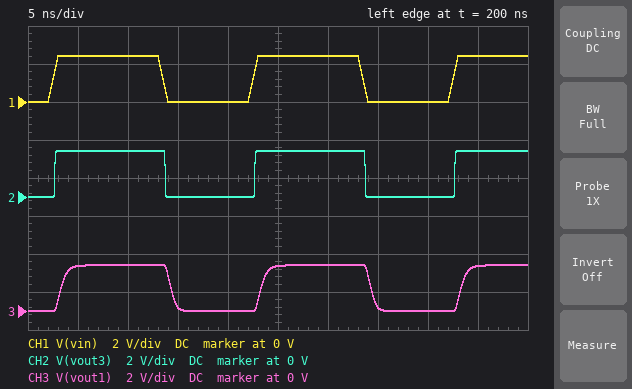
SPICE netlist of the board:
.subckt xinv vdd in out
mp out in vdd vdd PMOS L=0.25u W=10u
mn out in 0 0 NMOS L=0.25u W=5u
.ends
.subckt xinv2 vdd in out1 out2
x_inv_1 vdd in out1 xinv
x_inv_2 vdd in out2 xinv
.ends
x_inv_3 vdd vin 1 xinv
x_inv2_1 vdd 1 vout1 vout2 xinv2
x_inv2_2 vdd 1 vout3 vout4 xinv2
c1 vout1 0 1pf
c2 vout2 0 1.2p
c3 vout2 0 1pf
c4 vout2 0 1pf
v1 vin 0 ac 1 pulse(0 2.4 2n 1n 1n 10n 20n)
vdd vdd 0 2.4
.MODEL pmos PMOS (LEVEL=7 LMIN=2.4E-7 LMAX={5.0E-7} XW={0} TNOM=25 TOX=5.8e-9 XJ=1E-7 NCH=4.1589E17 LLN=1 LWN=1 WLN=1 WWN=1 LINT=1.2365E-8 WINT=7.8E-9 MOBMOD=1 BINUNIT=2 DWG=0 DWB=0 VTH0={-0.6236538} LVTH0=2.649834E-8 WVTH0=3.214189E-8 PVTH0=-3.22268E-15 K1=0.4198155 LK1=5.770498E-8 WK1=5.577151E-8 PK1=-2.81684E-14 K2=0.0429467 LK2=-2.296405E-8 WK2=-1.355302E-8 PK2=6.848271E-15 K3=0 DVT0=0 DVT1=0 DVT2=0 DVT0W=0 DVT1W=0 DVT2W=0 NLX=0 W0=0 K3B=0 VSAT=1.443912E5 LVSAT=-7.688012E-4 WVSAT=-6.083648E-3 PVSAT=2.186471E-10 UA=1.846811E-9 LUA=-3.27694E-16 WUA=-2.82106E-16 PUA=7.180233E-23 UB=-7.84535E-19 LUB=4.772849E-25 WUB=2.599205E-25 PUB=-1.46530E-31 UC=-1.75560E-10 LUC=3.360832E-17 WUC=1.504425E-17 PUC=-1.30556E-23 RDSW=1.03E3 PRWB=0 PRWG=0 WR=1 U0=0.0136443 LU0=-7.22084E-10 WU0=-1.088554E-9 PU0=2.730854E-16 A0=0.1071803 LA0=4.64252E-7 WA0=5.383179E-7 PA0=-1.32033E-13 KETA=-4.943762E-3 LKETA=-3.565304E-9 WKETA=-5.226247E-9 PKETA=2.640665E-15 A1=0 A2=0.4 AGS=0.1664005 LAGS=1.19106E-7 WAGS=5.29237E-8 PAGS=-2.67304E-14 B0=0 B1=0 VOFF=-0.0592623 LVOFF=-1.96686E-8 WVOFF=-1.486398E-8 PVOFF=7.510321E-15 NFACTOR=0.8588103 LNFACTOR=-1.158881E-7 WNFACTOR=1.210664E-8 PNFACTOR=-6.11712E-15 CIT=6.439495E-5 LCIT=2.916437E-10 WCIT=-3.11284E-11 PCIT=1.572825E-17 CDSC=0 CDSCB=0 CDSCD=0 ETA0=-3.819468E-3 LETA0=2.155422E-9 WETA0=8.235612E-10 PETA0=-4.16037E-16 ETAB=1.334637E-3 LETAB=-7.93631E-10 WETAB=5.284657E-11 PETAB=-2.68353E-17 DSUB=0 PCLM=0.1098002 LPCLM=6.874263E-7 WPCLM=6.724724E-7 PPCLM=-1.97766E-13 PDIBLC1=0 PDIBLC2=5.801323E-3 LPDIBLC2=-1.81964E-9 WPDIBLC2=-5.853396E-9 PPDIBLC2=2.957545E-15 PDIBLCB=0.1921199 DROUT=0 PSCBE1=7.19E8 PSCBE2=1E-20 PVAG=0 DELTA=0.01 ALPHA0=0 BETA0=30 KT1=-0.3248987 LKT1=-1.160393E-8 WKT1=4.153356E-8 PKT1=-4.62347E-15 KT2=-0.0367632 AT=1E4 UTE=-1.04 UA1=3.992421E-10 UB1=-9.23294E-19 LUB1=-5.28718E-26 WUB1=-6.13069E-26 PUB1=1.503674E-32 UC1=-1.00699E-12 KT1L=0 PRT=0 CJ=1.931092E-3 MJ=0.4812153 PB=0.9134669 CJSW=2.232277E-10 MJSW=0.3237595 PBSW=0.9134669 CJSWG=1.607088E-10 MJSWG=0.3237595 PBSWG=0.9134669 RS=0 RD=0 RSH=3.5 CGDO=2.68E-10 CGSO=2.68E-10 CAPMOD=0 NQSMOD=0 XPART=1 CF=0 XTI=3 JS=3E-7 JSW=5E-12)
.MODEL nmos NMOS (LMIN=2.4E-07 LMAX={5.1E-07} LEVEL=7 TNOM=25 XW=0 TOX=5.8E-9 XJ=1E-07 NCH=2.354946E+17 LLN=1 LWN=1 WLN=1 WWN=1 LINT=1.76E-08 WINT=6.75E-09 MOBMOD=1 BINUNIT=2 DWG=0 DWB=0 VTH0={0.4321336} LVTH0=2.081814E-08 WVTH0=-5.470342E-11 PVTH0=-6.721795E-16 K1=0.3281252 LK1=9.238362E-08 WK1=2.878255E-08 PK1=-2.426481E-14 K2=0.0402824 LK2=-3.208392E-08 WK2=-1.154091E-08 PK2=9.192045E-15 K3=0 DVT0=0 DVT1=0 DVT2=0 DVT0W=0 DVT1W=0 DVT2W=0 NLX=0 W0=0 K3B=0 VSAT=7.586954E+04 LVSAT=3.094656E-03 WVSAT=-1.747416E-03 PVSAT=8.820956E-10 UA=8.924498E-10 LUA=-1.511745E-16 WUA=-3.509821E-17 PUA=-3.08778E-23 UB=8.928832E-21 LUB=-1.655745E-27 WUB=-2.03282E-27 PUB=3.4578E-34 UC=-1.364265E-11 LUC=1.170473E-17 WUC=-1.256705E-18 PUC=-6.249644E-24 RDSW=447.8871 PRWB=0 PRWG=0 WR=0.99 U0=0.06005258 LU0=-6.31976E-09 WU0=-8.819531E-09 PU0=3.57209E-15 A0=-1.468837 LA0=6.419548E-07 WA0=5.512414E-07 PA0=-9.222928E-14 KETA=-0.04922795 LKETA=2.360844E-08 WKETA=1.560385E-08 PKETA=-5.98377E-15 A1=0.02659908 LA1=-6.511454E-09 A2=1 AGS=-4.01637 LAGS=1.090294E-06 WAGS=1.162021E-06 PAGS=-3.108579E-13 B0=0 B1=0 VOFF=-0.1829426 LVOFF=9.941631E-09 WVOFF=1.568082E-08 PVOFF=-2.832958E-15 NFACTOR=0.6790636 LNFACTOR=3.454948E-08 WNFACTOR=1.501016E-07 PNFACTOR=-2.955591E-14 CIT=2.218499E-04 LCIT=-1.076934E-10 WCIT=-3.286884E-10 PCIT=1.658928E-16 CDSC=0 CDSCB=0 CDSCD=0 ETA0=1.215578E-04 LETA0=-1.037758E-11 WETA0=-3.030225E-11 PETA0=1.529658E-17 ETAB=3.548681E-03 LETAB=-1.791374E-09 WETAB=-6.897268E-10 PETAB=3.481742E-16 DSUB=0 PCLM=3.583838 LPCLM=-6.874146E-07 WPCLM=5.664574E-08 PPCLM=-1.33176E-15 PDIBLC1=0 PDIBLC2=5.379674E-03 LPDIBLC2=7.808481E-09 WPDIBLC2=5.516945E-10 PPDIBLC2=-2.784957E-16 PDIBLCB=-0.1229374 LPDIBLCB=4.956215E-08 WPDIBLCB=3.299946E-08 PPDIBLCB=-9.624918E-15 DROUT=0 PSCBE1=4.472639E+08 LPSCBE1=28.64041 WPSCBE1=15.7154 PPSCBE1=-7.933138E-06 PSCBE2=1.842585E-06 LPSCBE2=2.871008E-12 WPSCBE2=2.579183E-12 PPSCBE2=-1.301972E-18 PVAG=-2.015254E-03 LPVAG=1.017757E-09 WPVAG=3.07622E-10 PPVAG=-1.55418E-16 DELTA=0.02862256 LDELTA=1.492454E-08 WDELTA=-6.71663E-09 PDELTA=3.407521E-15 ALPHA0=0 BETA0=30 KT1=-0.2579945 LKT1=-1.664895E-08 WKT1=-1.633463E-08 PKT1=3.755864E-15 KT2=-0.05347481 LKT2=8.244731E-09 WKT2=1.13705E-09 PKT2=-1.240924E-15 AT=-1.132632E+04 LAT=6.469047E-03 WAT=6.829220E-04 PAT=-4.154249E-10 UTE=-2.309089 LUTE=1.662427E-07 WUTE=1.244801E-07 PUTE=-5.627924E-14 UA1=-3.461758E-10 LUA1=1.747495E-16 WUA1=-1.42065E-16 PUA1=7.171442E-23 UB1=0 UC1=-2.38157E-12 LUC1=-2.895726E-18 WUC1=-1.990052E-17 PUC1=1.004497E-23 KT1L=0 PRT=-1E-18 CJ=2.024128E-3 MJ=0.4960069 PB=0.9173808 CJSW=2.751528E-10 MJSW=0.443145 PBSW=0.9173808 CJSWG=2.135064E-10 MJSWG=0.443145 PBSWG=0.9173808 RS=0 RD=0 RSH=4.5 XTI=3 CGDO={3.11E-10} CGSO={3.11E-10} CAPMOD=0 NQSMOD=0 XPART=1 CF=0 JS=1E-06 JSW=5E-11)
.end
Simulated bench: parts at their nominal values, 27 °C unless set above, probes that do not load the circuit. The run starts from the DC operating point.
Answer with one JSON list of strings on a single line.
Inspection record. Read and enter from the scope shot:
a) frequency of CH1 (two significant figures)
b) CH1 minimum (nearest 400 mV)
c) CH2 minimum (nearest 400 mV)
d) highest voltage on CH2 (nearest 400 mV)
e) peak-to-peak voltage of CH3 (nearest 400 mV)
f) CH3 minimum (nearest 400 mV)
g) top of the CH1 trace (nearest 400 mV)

["50 MHz", "0 V", "0 V", "2.4 V", "2.4 V", "0 V", "2.4 V"]
